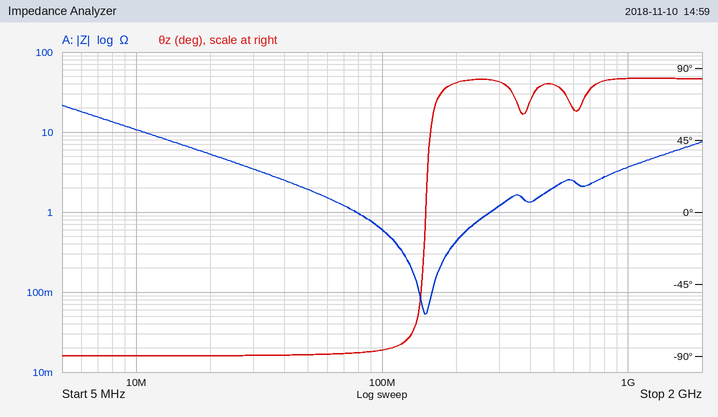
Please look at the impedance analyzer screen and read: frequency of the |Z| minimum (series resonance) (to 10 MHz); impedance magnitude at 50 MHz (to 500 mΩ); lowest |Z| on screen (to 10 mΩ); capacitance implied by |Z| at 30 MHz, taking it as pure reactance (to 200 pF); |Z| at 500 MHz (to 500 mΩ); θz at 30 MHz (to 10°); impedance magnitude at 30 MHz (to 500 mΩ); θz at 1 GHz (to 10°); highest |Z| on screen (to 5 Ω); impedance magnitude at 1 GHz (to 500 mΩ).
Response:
150 MHz
2.0 Ω
50 mΩ
1.6 nF
2.0 Ω
-90°
3.5 Ω
80°
20 Ω
3.5 Ω
